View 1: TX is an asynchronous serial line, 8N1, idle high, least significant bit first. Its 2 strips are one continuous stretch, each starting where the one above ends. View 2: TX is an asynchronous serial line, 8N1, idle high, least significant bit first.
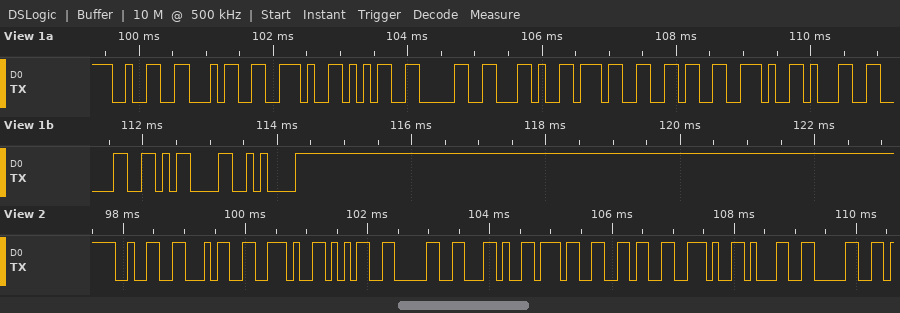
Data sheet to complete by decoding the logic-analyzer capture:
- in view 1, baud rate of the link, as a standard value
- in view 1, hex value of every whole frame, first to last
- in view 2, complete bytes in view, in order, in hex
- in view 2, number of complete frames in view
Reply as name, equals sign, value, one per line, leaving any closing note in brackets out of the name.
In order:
in view 1, baud rate of the link, as a standard value = 9600 baud
in view 1, hex value of every whole frame, first to last = 32 34 2E 35 30 2C 37 36 2E 31 30 0D 0A
in view 2, complete bytes in view, in order, in hex = 32 34 2E 35 30 2C 37 36 2E 31 30
in view 2, number of complete frames in view = 11
